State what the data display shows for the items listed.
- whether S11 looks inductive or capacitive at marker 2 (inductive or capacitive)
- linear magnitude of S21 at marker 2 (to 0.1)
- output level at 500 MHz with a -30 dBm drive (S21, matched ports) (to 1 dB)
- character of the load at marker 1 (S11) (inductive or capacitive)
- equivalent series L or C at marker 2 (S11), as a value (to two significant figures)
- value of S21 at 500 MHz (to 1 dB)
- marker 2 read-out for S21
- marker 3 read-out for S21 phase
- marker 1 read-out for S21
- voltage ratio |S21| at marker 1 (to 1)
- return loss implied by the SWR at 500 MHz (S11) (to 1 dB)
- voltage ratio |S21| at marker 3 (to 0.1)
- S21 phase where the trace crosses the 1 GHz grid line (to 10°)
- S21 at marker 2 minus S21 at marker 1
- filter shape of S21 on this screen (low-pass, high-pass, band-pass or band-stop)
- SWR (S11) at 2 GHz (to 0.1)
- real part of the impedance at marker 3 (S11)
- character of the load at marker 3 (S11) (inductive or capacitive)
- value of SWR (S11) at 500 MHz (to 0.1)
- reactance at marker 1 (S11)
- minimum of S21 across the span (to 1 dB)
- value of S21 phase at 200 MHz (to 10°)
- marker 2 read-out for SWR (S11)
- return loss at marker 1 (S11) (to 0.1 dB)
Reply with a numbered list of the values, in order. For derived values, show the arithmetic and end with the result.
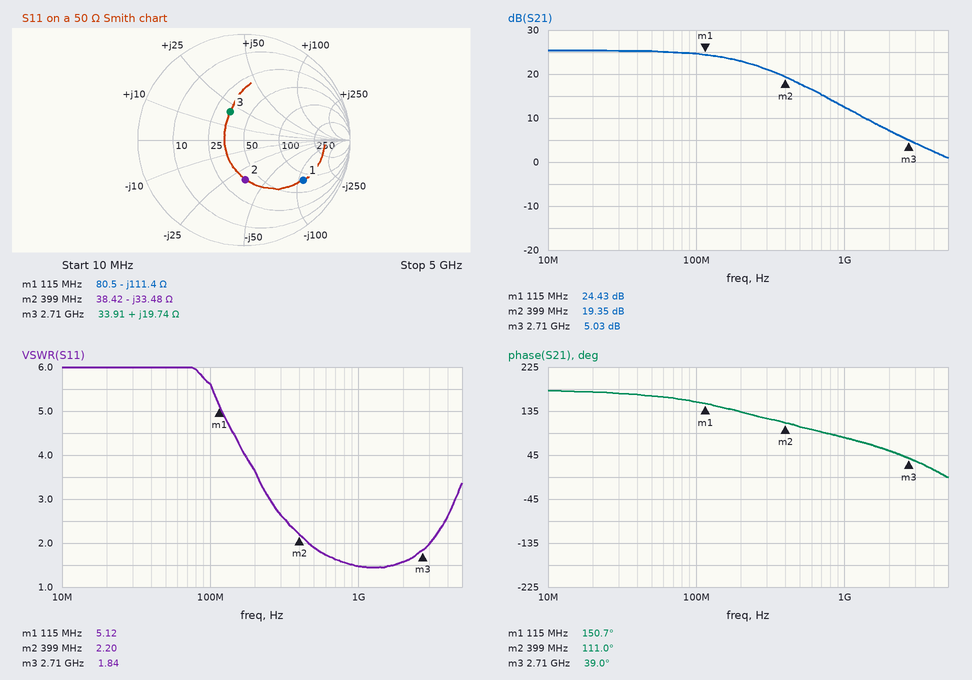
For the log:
1. capacitive
2. 10^(19.35/20) ≈ 9.3
3. -30 dBm + (18 dB) = -12 dBm
4. capacitive
5. C = 1/(2π × 399 MHz × 33.48 Ω) ≈ 12 pF
6. 18 dB
7. 19.35 dB
8. 39.0°
9. 24.43 dB
10. 10^(24.43/20) ≈ 17
11. −20 log10((1.9 − 1)/(1.9 + 1)) ≈ 10 dB
12. 10^(5.03/20) ≈ 1.8
13. 80°
14. 19.35 − (24.43) = -5.08 dB
15. low-pass
16. 1.6
17. 33.91 Ω
18. inductive
19. 1.9
20. -111.4 Ω
21. 1 dB
22. 130°
23. 2.20
24. 3.4 dB
